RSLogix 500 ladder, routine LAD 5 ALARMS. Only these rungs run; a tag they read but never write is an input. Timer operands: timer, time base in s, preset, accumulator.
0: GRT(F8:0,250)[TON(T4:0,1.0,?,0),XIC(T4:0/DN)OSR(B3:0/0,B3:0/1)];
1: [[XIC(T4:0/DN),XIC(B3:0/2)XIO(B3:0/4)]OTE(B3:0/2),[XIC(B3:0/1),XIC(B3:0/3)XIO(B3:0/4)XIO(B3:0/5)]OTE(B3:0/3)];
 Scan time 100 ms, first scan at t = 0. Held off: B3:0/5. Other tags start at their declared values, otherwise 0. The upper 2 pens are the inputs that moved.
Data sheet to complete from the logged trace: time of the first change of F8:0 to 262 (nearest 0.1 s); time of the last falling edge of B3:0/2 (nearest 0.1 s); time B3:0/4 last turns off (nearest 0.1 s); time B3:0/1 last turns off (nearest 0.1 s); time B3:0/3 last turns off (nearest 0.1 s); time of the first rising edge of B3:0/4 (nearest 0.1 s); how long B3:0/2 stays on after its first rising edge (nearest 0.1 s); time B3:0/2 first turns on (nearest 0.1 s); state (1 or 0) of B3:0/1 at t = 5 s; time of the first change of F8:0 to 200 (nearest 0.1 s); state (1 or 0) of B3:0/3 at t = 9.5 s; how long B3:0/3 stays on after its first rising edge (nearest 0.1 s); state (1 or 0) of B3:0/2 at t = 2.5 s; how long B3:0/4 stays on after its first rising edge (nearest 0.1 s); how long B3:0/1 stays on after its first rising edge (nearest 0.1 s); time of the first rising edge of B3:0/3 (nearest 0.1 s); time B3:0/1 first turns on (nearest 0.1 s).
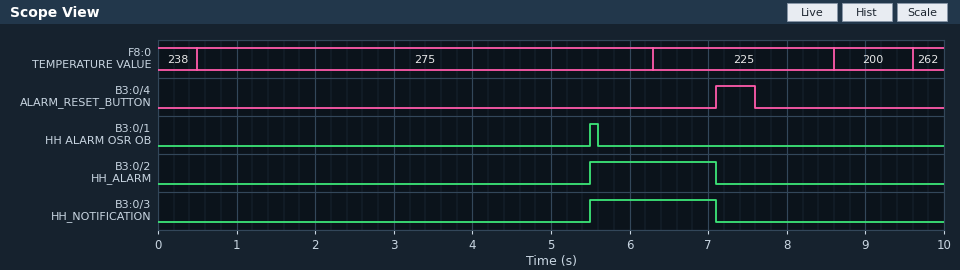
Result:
9.6 s
7.1 s
7.6 s
5.6 s
7.1 s
7.1 s
1.6 s
5.5 s
0
8.6 s
0
1.6 s
0
0.5 s
0.1 s
5.5 s
5.5 s
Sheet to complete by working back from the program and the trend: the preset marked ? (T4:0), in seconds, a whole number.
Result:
5 s
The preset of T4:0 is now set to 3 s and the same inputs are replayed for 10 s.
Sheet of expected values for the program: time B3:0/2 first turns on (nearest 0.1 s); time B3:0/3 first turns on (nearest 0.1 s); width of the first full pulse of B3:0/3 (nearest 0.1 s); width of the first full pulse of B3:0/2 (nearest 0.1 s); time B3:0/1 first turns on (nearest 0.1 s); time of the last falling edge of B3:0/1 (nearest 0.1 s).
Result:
3.5 s
3.5 s
3.6 s
3.6 s
3.5 s
3.6 s
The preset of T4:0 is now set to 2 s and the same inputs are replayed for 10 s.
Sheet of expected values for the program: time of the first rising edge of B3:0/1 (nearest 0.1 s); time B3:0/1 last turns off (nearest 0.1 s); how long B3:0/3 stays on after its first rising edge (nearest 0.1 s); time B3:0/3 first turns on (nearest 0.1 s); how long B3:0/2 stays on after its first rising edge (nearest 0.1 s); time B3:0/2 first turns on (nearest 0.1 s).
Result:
2.5 s
2.6 s
4.6 s
2.5 s
4.6 s
2.5 s
